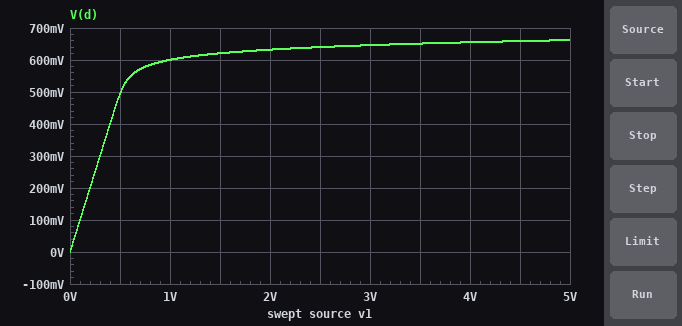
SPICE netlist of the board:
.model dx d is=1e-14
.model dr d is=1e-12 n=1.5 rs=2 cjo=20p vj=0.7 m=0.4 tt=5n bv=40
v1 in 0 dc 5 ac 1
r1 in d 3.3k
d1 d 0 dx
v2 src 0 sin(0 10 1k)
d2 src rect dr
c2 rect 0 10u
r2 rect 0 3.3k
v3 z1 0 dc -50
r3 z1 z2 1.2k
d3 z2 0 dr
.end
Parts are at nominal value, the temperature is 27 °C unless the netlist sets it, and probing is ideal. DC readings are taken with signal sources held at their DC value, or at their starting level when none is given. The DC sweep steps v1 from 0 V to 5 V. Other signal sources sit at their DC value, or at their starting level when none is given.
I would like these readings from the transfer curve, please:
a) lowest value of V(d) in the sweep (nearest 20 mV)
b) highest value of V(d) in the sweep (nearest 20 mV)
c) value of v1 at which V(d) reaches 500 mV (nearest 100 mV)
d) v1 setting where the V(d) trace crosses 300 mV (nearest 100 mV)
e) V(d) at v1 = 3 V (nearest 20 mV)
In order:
0 V
660 mV
500 mV
300 mV
640 mV
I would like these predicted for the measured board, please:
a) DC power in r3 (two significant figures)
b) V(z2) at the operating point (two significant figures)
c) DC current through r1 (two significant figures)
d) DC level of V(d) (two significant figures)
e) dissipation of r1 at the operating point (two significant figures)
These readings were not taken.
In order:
82 mW
-40 V
1.3 mA
660 mV
5.7 mW
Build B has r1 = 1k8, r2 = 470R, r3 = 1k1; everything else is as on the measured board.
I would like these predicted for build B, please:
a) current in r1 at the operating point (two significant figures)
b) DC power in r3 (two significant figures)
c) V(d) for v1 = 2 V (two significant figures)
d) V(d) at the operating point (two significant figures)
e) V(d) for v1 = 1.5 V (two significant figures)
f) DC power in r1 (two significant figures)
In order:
2.4 mA
89 mW
650 mV
680 mV
640 mV
10 mW
